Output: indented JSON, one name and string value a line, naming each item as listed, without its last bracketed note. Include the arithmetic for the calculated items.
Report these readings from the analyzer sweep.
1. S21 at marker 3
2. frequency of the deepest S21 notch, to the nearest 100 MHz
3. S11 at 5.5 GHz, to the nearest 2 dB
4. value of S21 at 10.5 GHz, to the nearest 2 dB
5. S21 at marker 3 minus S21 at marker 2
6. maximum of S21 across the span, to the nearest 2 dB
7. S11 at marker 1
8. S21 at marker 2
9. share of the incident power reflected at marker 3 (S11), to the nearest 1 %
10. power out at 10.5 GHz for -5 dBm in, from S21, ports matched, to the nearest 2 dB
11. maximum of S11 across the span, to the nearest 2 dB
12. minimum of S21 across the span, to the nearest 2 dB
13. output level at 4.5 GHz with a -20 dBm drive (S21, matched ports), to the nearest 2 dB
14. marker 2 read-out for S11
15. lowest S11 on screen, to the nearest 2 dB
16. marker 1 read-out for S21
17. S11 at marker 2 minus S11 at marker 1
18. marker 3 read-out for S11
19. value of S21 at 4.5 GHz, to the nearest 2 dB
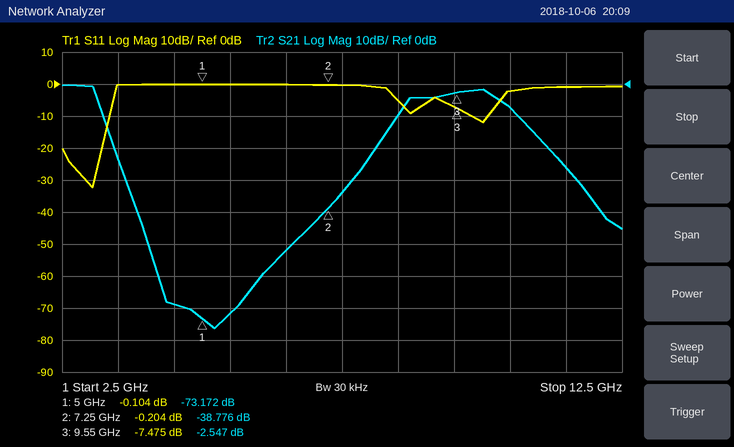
{
  "S21 at marker 3": "-2.547 dB",
  "frequency of the deepest S21 notch, to the nearest 100 MHz": "5.2 GHz",
  "S11 at 5.5 GHz, to the nearest 2 dB": "0 dB",
  "value of S21 at 10.5 GHz, to the nearest 2 dB": "-8 dB",
  "S21 at marker 3 minus S21 at marker 2": "-2.547 − (-38.776) = 36.229 dB",
  "maximum of S21 across the span, to the nearest 2 dB": "0 dB",
  "S11 at marker 1": "-0.104 dB",
  "S21 at marker 2": "-38.776 dB",
  "share of the incident power reflected at marker 3 (S11), to the nearest 1 %": "10^(-7.475/10) ≈ 18 %",
  "power out at 10.5 GHz for -5 dBm in, from S21, ports matched, to the nearest 2 dB": "-5 dBm + (-8 dB) = -12 dBm",
  "maximum of S11 across the span, to the nearest 2 dB": "0 dB",
  "minimum of S21 across the span, to the nearest 2 dB": "-76 dB",
  "output level at 4.5 GHz with a -20 dBm drive (S21, matched ports), to the nearest 2 dB": "-20 dBm + (-68 dB) = -88 dBm",
  "marker 2 read-out for S11": "-0.204 dB",
  "lowest S11 on screen, to the nearest 2 dB": "-32 dB",
  "marker 1 read-out for S21": "-73.172 dB",
  "S11 at marker 2 minus S11 at marker 1": "-0.204 − (-0.104) = -0.100 dB",
  "marker 3 read-out for S11": "-7.475 dB",
  "value of S21 at 4.5 GHz, to the nearest 2 dB": "-68 dB"
}
